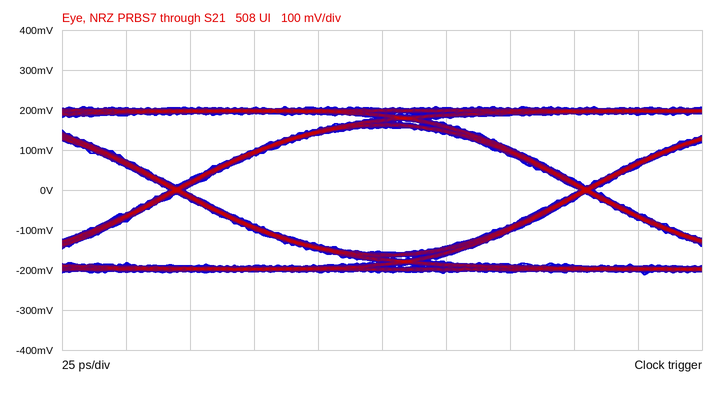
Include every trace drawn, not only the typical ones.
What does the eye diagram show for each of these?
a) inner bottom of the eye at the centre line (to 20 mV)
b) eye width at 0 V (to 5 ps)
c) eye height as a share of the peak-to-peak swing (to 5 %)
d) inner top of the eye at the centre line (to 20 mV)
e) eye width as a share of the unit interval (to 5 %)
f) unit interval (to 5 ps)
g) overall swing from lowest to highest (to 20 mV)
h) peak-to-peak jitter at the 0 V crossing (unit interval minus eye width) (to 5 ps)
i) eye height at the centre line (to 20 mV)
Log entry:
-160 mV
155 ps
75 %
160 mV
95 %
160 ps
420 mV
5 ps
320 mV
